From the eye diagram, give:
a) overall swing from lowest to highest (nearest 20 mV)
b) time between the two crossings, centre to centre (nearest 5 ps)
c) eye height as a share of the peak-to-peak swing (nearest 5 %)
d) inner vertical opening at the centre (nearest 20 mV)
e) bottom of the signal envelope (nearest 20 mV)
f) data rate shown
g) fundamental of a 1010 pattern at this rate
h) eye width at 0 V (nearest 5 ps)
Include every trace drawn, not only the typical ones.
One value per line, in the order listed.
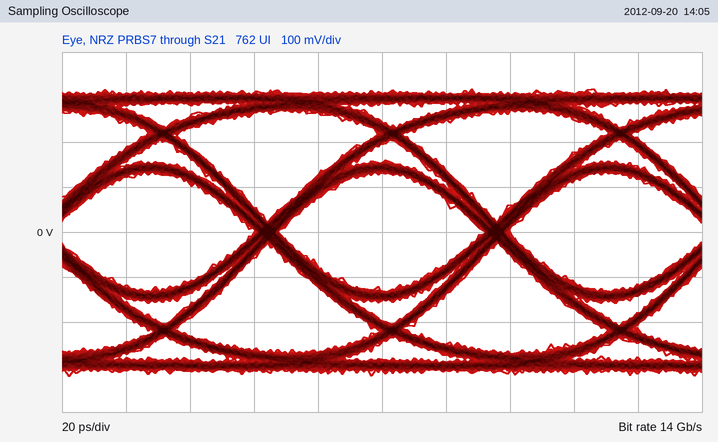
640 mV
70 ps
40 %
260 mV
-320 mV
14 Gb/s
7 GHz
65 ps
